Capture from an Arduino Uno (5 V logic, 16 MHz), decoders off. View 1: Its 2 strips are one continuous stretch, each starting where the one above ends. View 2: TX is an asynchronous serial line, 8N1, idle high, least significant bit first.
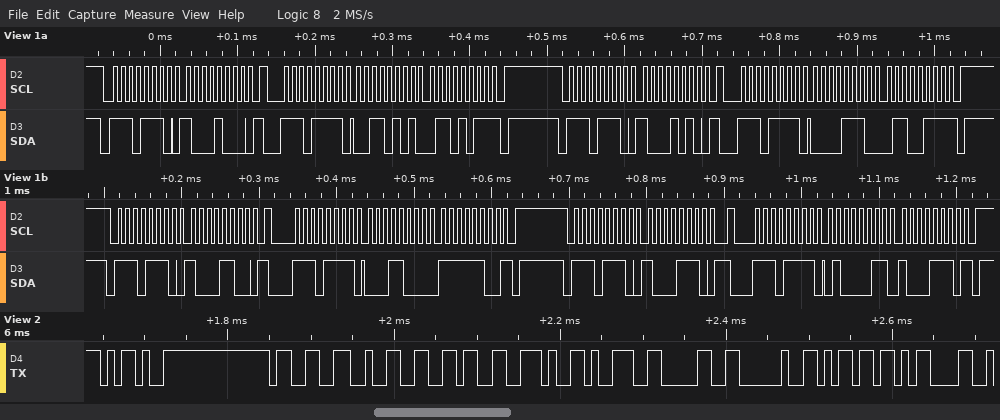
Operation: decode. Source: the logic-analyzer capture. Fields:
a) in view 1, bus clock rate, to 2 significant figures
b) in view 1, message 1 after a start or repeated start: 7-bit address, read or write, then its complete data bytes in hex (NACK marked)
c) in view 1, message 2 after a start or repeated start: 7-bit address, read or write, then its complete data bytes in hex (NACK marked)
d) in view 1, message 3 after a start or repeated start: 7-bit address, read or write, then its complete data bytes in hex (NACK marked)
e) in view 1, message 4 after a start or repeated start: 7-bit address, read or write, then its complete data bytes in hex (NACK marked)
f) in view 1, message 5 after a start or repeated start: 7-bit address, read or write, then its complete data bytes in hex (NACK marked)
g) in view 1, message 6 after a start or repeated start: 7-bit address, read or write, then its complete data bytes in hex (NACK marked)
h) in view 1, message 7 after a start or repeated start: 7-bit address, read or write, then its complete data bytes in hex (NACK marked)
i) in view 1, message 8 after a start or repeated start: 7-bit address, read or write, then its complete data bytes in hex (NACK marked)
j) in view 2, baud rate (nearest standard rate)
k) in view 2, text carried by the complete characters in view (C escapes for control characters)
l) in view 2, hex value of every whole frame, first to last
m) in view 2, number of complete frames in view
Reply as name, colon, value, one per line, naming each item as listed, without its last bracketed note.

in view 1, bus clock rate, to 2 significant figures: 100 kHz
in view 1, message 1 after a start or repeated start: 7-bit address, read or write, then its complete data bytes in hex: 0x77 write: 88
in view 1, message 2 after a start or repeated start: 7-bit address, read or write, then its complete data bytes in hex: 0x77 read: 35 6B NACK
in view 1, message 3 after a start or repeated start: 7-bit address, read or write, then its complete data bytes in hex: 0x77 write: 8A
in view 1, message 4 after a start or repeated start: 7-bit address, read or write, then its complete data bytes in hex: 0x77 read: 0E 67 NACK
in view 1, message 5 after a start or repeated start: 7-bit address, read or write, then its complete data bytes in hex: 0x77 write: 8C
in view 1, message 6 after a start or repeated start: 7-bit address, read or write, then its complete data bytes in hex: 0x77 read: 18 FC NACK
in view 1, message 7 after a start or repeated start: 7-bit address, read or write, then its complete data bytes in hex: 0x77 write: 8E
in view 1, message 8 after a start or repeated start: 7-bit address, read or write, then its complete data bytes in hex: 0x77 read: 43 8E NACK
in view 2, baud rate: 115200 baud
in view 2, text carried by the complete characters in view: "-326.90 m\r"
in view 2, hex value of every whole frame, first to last: 0x2D 0x33 0x32 0x36 0x2E 0x39 0x30 0x20 0x6D 0x0D
in view 2, number of complete frames in view: 10
